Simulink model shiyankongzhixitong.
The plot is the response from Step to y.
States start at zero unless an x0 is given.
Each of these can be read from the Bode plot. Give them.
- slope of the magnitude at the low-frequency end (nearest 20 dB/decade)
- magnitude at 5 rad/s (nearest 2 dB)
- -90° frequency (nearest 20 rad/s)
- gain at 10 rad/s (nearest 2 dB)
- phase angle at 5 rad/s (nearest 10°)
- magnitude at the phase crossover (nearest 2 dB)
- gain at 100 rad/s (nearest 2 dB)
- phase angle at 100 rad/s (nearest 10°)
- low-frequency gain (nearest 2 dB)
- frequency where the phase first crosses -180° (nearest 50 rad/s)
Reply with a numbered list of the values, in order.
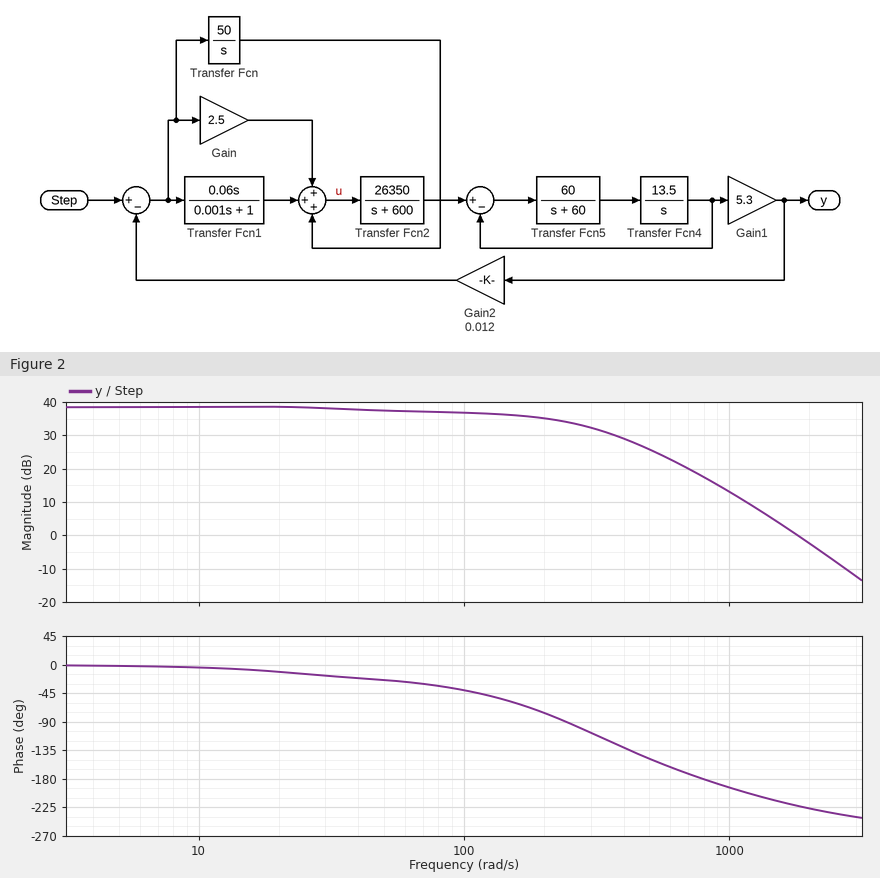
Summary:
1. 0 dB/decade
2. 38 dB
3. 240 rad/s
4. 38 dB
5. 0°
6. 18 dB
7. 36 dB
8. -40°
9. 38 dB
10. 800 rad/s
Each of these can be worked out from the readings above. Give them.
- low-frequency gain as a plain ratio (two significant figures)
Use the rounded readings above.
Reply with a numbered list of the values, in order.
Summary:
1. 79
